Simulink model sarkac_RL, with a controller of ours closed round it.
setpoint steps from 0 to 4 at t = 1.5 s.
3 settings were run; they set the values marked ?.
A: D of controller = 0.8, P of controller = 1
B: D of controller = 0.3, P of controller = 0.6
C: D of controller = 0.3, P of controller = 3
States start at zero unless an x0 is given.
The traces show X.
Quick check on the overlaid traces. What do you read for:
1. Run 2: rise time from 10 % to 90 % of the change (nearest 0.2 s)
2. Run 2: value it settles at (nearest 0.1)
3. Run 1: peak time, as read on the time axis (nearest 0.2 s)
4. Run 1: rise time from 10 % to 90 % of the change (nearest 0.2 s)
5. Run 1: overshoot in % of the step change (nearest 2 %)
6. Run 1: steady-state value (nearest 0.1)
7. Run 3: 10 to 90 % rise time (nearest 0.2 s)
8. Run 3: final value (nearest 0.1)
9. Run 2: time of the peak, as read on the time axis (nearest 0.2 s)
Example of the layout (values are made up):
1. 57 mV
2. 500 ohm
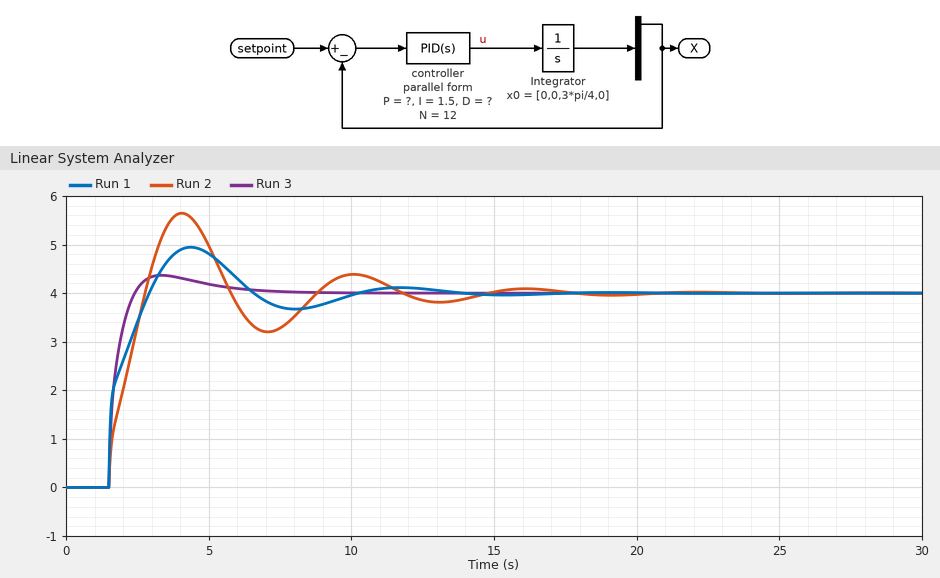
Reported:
1. 1.0 s
2. 4.0
3. 4.4 s
4. 1.2 s
5. 24 %
6. 4.0
7. 0.6 s
8. 4.0
9. 4.0 s
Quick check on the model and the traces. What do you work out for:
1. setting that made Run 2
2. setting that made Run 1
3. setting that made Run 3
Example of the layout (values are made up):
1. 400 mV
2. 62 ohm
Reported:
1. B
2. A
3. C
